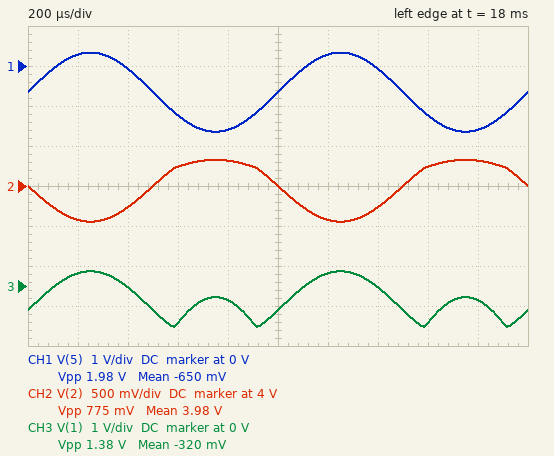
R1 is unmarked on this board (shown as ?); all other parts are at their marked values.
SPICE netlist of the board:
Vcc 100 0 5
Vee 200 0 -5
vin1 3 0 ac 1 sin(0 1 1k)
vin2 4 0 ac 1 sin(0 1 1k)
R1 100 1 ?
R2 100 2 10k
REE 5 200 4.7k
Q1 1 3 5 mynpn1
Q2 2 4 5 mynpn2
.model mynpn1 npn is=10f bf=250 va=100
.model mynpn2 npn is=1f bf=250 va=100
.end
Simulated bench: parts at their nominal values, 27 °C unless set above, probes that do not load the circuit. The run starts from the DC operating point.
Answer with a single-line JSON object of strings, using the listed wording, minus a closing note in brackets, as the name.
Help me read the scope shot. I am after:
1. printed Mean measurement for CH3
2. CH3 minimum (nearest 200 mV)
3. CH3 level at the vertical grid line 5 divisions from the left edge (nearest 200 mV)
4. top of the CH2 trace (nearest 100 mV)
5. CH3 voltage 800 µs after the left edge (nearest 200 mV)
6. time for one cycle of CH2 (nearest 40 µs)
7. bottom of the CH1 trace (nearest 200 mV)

{"printed Mean measurement for CH3": "-320 mV", "CH3 minimum": "-1.0 V", "CH3 level at the vertical grid line 5 divisions from the left edge": "-600 mV", "top of the CH2 trace": "4.3 V", "CH3 voltage 800 µs after the left edge": "-400 mV", "time for one cycle of CH2": "1.00 ms", "bottom of the CH1 trace": "-1.6 V"}
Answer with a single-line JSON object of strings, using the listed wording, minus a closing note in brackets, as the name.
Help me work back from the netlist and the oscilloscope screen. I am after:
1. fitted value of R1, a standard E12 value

{"fitted value of R1, a standard E12 value": "8.2 kΩ"}
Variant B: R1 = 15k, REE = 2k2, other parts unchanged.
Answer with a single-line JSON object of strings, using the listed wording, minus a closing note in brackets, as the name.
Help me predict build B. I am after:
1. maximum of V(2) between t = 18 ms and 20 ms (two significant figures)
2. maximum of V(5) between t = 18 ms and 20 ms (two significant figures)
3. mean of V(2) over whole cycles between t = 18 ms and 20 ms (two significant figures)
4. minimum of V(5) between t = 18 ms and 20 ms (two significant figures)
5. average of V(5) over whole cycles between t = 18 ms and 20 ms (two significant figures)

{"maximum of V(2) between t = 18 ms and 20 ms": "2.8 V", "maximum of V(5) between t = 18 ms and 20 ms": "310 mV", "mean of V(2) over whole cycles between t = 18 ms and 20 ms": "2.0 V", "minimum of V(5) between t = 18 ms and 20 ms": "-1.7 V", "average of V(5) over whole cycles between t = 18 ms and 20 ms": "-680 mV"}
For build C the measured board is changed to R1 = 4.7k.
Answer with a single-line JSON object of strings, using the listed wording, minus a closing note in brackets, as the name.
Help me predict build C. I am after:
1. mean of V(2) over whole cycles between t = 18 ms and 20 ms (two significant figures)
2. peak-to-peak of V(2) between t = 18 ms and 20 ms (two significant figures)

{"mean of V(2) over whole cycles between t = 18 ms and 20 ms": "4.1 V", "peak-to-peak of V(2) between t = 18 ms and 20 ms": "450 mV"}
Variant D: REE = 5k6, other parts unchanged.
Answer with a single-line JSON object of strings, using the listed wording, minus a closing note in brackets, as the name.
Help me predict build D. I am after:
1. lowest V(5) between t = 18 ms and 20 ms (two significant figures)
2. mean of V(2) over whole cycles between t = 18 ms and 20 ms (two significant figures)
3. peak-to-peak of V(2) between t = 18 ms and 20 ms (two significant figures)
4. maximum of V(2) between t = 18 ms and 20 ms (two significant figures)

{"lowest V(5) between t = 18 ms and 20 ms": "-1.6 V", "mean of V(2) over whole cycles between t = 18 ms and 20 ms": "4.2 V", "peak-to-peak of V(2) between t = 18 ms and 20 ms": "580 mV", "maximum of V(2) between t = 18 ms and 20 ms": "4.4 V"}
